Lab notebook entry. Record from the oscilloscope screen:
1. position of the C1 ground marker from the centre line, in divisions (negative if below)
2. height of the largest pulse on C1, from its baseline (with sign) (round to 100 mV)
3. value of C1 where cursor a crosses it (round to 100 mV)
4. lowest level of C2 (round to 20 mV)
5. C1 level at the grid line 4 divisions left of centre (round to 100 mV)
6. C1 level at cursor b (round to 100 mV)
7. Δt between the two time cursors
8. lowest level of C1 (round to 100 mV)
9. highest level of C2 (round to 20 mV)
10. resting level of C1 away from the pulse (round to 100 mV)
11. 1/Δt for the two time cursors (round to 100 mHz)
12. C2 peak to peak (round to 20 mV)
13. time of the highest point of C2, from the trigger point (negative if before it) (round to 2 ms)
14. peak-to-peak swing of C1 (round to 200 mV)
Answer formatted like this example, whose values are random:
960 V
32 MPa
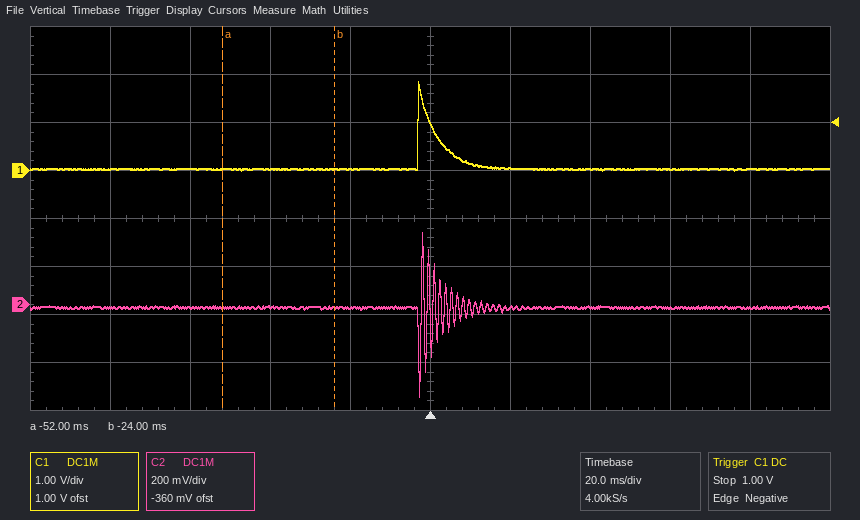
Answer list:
+1.0 div
+1.8 V
0.0 V
-380 mV
0.0 V
0.0 V
28 ms
0.0 V
300 mV
0.0 V
35.7 Hz
680 mV
-2 ms
1.8 V
